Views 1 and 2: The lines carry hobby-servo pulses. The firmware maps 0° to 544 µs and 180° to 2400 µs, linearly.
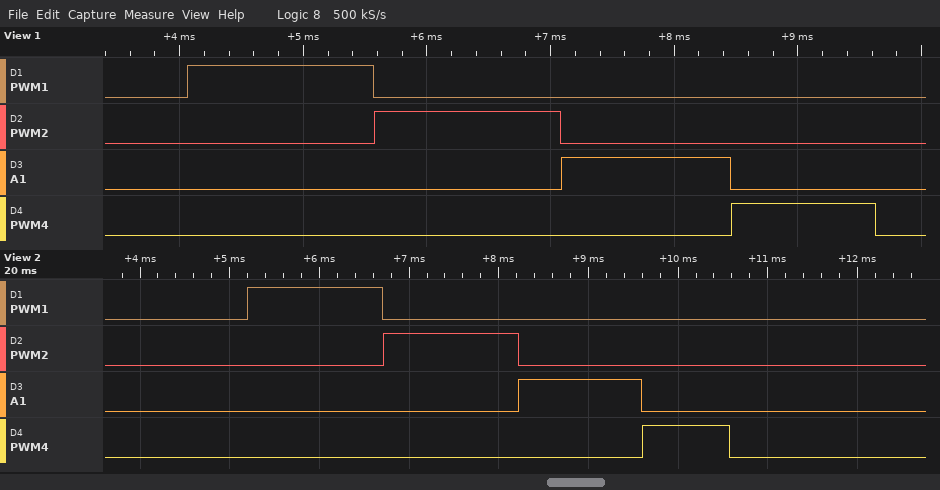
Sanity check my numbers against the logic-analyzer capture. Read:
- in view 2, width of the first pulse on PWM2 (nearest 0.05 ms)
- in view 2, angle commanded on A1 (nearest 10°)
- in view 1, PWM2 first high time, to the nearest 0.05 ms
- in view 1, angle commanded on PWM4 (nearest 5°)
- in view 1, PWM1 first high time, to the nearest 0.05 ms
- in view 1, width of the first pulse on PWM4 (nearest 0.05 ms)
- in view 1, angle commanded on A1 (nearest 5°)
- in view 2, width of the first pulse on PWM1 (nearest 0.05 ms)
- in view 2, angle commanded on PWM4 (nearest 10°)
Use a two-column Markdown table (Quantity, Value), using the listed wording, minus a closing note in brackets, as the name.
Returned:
| Quantity | Value |
|---|---|
| in view 2, width of the first pulse on PWM2 | 1.50 ms |
| in view 2, angle commanded on A1 | 80° |
| in view 1, PWM2 first high time, to the nearest 0.05 ms | 1.50 ms |
| in view 1, angle commanded on PWM4 | 60° |
| in view 1, PWM1 first high time, to the nearest 0.05 ms | 1.50 ms |
| in view 1, width of the first pulse on PWM4 | 1.15 ms |
| in view 1, angle commanded on A1 | 80° |
| in view 2, width of the first pulse on PWM1 | 1.50 ms |
| in view 2, angle commanded on PWM4 | 40° |
